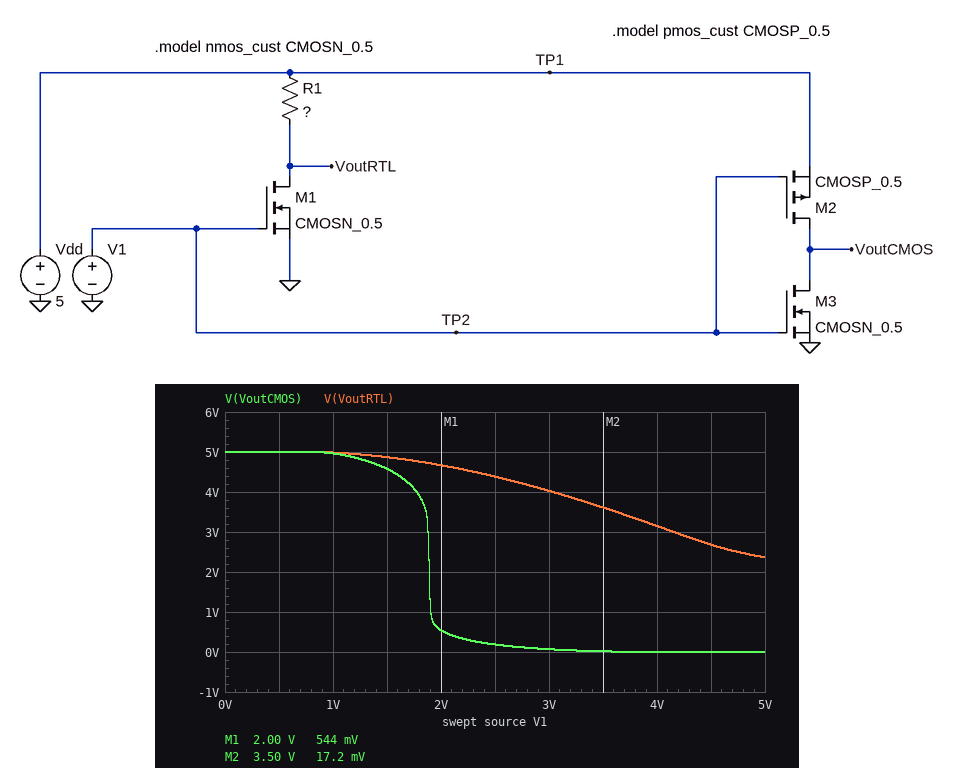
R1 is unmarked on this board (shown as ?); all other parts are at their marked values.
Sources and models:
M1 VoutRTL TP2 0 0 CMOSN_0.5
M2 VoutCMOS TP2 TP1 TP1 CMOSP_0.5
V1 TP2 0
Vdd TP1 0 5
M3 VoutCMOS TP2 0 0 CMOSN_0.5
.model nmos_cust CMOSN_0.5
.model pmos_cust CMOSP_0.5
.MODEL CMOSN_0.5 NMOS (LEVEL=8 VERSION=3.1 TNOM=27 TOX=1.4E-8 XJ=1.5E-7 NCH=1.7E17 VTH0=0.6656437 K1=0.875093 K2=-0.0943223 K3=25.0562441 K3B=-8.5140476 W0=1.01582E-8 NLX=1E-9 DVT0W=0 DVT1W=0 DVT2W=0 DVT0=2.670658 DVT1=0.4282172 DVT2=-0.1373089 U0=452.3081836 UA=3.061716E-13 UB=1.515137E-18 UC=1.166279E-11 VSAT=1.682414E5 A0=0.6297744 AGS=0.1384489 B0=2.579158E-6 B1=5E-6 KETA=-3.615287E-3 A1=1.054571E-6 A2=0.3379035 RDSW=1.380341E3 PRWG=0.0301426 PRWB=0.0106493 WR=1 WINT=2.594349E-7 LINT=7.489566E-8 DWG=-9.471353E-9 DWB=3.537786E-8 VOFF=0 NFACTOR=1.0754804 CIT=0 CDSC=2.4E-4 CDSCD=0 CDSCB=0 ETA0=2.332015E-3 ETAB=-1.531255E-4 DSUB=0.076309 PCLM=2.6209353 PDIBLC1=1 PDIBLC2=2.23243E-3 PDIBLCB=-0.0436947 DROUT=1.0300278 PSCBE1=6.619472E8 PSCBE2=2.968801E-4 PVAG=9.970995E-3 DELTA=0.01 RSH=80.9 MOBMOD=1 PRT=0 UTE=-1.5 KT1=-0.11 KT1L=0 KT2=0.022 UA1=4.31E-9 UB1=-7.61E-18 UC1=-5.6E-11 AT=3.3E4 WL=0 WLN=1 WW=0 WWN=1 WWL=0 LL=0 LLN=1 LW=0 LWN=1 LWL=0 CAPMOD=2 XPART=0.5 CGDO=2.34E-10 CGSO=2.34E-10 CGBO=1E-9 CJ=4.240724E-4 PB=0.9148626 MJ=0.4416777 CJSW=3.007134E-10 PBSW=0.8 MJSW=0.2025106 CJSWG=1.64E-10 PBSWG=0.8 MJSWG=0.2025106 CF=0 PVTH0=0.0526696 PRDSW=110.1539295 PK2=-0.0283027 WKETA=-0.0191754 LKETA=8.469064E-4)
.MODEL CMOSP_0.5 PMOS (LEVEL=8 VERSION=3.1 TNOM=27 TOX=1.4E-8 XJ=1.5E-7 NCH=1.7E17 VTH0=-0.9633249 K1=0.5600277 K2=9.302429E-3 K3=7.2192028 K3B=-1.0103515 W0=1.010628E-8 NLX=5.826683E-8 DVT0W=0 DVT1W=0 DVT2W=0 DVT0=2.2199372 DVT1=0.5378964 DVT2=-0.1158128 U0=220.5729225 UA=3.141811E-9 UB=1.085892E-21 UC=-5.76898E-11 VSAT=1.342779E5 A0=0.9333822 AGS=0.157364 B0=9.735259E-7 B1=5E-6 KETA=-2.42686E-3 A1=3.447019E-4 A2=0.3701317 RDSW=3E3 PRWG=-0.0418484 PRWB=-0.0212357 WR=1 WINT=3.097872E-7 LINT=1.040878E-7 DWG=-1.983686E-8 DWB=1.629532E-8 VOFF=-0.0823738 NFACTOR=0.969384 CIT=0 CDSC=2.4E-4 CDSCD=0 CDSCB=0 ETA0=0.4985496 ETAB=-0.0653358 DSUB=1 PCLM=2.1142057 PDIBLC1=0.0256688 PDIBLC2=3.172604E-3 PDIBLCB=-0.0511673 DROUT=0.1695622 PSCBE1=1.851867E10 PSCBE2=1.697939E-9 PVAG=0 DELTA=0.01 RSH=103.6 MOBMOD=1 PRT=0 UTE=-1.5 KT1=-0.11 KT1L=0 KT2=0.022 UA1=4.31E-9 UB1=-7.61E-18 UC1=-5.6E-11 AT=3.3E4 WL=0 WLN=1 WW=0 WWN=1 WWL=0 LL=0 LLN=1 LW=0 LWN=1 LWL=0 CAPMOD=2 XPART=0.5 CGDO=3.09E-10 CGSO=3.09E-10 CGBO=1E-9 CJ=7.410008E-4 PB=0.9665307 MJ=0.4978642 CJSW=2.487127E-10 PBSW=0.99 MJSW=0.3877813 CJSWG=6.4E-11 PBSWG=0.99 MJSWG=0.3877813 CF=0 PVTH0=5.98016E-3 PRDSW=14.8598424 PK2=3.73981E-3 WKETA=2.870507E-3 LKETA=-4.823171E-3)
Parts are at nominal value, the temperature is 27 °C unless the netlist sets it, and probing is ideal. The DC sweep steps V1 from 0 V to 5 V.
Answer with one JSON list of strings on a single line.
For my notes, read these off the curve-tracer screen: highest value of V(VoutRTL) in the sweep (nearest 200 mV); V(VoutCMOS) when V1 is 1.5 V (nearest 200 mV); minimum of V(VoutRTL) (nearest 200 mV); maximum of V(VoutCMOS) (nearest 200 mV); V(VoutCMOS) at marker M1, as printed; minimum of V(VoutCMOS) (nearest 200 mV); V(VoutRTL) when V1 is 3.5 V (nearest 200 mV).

["5.0 V", "4.6 V", "2.4 V", "5.0 V", "544 mV", "0 V", "3.6 V"]
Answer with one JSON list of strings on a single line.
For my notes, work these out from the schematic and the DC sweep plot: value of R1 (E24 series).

["5.6 kΩ"]
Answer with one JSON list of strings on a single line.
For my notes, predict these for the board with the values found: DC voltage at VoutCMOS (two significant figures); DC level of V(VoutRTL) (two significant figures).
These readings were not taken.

["5.0 V", "5.0 V"]
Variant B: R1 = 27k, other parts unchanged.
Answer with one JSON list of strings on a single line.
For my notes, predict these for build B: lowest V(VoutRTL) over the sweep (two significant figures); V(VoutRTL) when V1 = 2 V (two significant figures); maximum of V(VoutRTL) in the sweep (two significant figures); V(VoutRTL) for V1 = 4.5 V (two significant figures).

["590 mV", "3.4 V", "5.0 V", "650 mV"]
